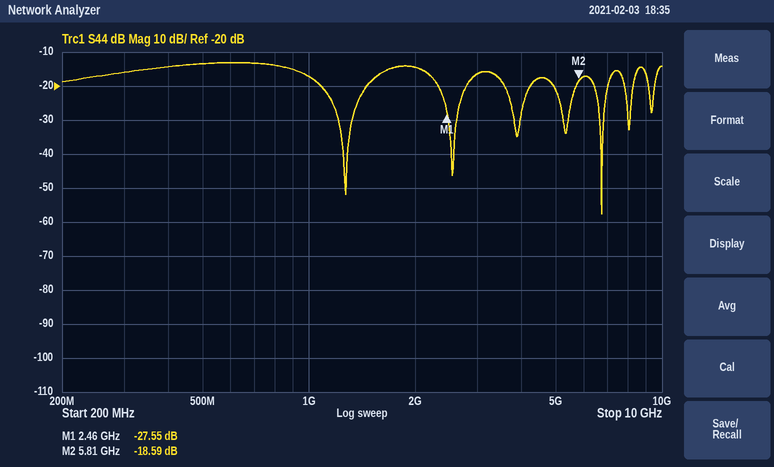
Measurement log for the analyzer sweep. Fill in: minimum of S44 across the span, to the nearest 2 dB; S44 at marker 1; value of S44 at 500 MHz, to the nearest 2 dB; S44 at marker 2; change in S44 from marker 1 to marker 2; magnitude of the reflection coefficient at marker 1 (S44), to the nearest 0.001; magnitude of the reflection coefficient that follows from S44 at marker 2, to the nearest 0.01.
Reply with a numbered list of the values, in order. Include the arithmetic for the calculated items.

1. -58 dB
2. -27.55 dB
3. -14 dB
4. -18.59 dB
5. -18.59 − (-27.55) = 8.96 dB
6. 10^(-27.55/20) ≈ 0.042
7. 10^(-18.59/20) ≈ 0.12
